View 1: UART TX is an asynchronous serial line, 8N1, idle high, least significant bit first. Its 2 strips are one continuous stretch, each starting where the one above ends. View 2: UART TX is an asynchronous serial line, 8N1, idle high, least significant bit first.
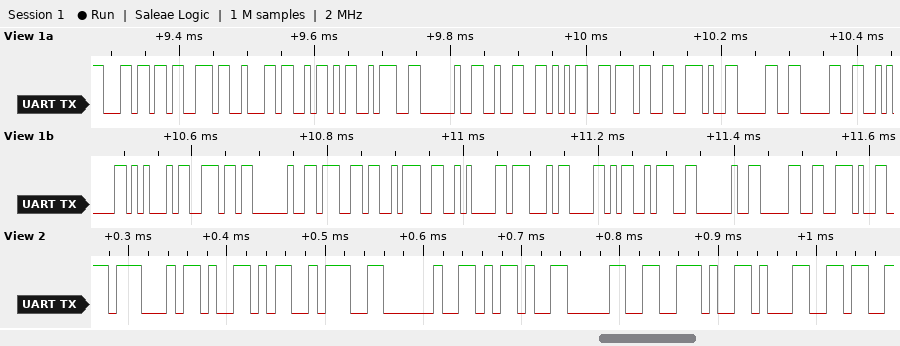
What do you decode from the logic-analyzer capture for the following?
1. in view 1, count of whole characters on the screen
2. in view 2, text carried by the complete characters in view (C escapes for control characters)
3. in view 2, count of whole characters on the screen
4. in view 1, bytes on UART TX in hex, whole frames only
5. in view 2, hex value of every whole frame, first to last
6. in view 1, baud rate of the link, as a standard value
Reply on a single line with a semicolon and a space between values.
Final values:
25; "GY: -0.1"; 8; 6C 73 62 5A 3A 20 32 35 37 2E 30 30 0A 45 6E 20 67 3A 0A 47 58 3A 20 30 2E; 47 59 3A 20 2D 30 2E 31; 115200 baud
